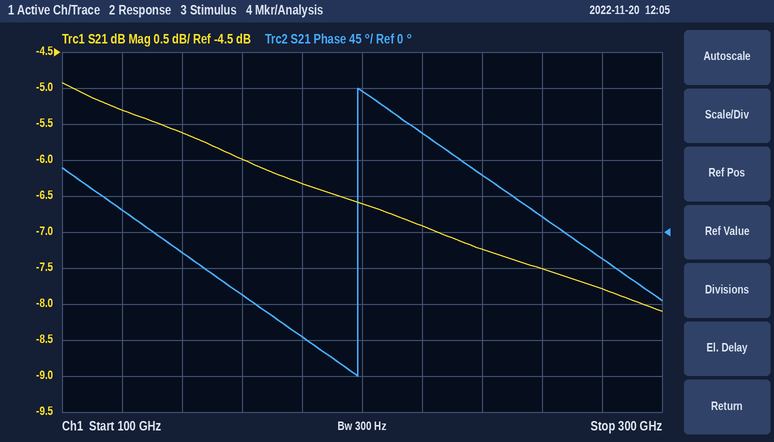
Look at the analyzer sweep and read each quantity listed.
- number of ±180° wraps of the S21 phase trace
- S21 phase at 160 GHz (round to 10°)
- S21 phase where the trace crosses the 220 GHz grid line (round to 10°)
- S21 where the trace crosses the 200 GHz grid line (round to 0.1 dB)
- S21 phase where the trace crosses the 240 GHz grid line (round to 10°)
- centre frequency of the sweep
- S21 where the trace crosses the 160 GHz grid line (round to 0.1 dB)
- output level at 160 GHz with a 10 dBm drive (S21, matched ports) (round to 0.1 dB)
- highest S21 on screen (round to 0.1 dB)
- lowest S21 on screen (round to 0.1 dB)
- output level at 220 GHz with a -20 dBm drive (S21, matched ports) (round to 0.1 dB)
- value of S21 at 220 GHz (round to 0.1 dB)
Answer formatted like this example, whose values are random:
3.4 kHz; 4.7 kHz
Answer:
1; -80°; 120°; -6.6 dB; 70°; 200 GHz; -6.0 dB; 4.0 dBm; -4.9 dB; -8.1 dB; -26.9 dBm; -6.9 dB
